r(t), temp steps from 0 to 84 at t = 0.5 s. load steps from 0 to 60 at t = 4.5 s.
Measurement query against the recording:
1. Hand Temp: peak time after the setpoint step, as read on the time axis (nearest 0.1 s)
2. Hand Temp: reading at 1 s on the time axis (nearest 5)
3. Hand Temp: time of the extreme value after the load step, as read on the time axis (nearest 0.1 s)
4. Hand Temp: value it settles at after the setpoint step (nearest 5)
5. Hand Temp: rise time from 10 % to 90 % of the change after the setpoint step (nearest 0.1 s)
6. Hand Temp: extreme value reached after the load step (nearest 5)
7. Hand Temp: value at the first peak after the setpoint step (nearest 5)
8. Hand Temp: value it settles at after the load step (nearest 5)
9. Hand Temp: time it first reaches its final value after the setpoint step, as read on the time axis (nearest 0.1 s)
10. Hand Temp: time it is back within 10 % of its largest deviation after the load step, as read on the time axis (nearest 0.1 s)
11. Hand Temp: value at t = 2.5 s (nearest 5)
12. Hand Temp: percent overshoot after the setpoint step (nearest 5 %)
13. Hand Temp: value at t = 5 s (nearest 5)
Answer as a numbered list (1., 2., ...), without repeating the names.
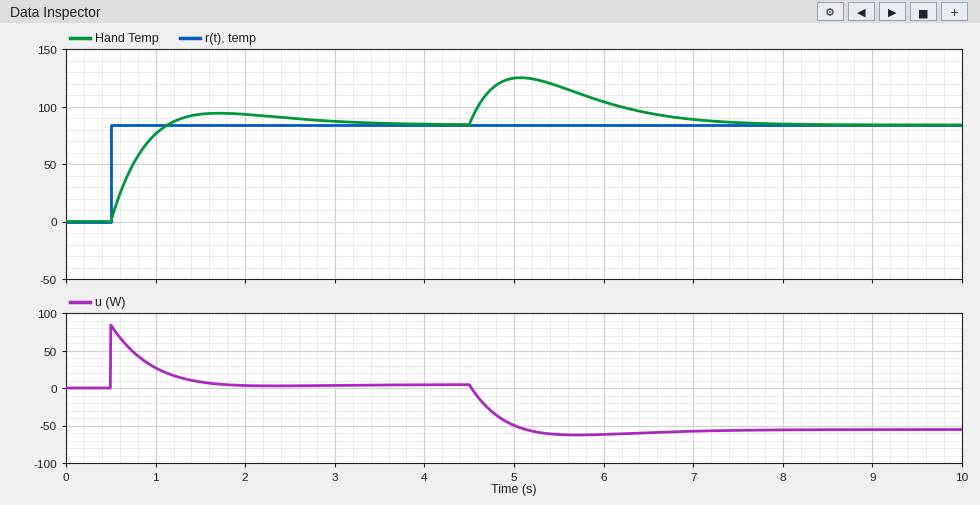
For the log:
1. 1.7 s
2. 75
3. 5.1 s
4. 85
5. 0.5 s
6. 125
7. 95
8. 85
9. 1.1 s
10. 7.1 s
11. 90
12. 10 %
13. 125
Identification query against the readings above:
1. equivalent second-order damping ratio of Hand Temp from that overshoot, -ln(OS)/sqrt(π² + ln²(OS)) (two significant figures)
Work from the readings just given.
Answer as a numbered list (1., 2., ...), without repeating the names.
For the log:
1. 0.59
